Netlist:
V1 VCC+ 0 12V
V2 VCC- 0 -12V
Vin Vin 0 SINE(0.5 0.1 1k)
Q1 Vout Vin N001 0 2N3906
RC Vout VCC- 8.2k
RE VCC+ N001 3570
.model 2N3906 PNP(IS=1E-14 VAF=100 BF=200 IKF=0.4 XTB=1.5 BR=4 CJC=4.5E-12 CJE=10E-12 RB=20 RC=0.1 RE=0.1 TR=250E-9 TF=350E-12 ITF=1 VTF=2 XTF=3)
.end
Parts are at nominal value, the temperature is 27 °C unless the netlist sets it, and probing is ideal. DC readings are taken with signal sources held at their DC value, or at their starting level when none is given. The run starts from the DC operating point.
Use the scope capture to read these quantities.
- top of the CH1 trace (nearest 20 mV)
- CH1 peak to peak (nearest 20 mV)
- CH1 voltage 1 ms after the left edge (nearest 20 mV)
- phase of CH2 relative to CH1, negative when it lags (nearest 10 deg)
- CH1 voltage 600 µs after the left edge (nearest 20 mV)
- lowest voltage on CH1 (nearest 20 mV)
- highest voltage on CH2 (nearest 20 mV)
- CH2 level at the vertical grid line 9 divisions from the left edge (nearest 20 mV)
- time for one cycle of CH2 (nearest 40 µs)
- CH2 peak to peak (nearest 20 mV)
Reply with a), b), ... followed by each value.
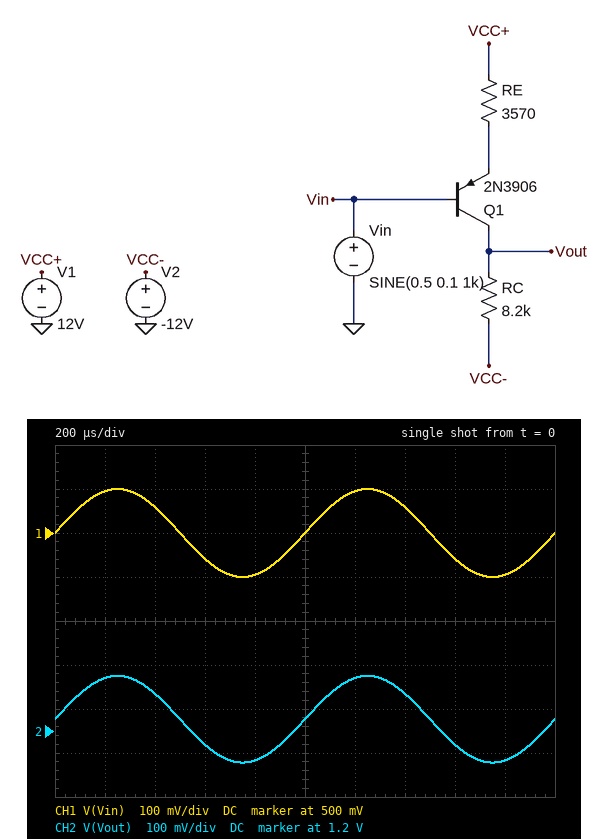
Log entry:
a) 600 mV
b) 200 mV
c) 500 mV
d) 0 deg
e) 440 mV
f) 400 mV
g) 1.32 V
h) 1.14 V
i) 1.00 ms
j) 200 mV
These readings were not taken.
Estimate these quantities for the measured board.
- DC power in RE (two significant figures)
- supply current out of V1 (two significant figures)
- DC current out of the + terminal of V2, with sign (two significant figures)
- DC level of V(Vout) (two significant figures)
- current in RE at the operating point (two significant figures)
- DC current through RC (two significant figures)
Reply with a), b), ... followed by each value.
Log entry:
a) 32 mW
b) 3.0 mA
c) -1.6 mA
d) 1.2 V
e) 3.0 mA
f) 1.6 mA
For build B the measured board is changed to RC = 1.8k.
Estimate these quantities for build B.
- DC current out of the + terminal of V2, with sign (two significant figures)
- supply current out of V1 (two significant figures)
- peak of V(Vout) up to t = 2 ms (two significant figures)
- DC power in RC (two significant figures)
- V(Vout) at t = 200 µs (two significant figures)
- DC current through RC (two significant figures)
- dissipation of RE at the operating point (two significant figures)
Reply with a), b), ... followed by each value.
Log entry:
a) -3.0 mA
b) 3.0 mA
c) -6.5 V
d) 16 mW
e) -6.6 V
f) 3.0 mA
g) 33 mW
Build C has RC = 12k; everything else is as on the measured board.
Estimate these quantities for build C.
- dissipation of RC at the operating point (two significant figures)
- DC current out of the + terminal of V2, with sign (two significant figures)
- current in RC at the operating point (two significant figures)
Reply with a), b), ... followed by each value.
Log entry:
a) 15 mW
b) -1.1 mA
c) 1.1 mA
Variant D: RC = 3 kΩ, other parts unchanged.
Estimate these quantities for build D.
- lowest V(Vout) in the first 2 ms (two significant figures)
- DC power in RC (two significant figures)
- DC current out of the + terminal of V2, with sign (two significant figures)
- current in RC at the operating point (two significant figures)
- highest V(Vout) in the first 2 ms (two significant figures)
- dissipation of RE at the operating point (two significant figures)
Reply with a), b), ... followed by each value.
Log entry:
a) -3.0 V
b) 27 mW
c) -3.0 mA
d) 3.0 mA
e) -2.9 V
f) 33 mW
